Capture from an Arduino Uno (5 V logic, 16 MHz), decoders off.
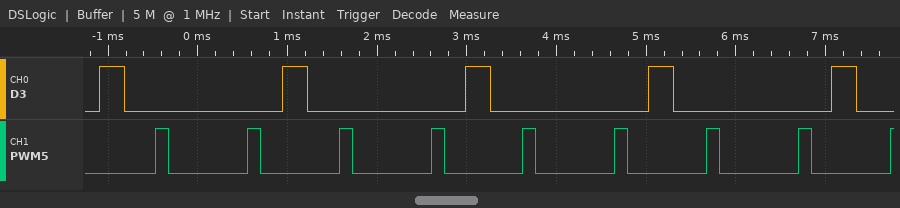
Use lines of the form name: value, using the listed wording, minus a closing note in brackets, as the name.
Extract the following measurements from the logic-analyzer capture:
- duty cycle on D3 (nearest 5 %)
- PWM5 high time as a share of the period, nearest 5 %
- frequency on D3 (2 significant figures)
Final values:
duty cycle on D3: 15 %
PWM5 high time as a share of the period, nearest 5 %: 15 %
frequency on D3: 490 Hz
